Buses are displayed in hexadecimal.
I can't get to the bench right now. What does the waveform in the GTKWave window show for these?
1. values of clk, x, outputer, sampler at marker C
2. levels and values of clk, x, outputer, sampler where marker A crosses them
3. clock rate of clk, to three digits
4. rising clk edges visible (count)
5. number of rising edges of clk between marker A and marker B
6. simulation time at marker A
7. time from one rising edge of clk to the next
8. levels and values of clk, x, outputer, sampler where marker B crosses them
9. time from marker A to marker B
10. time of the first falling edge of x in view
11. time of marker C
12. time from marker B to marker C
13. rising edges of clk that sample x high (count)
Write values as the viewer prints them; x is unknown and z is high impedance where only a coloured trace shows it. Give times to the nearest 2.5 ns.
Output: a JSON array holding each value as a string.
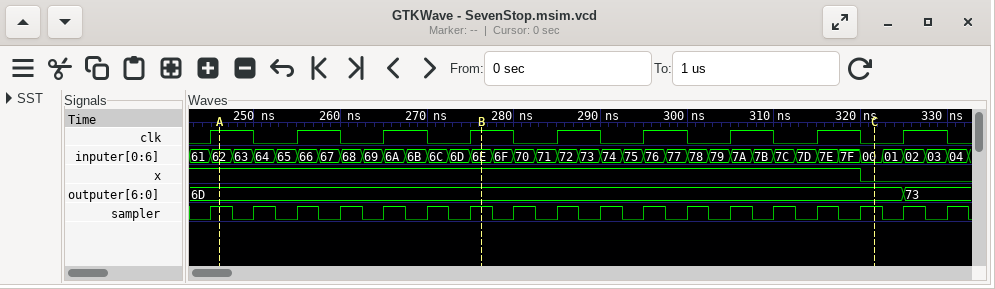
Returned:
["clk=0, x=0, outputer=6D, sampler=1", "clk=1, x=1, outputer=6D, sampler=1", "100 MHz", "9", "3", "245 ns", "10 ns", "clk=1, x=1, outputer=6D, sampler=1", "30 ns", "320 ns", "322.5 ns", "45 ns", "8"]
